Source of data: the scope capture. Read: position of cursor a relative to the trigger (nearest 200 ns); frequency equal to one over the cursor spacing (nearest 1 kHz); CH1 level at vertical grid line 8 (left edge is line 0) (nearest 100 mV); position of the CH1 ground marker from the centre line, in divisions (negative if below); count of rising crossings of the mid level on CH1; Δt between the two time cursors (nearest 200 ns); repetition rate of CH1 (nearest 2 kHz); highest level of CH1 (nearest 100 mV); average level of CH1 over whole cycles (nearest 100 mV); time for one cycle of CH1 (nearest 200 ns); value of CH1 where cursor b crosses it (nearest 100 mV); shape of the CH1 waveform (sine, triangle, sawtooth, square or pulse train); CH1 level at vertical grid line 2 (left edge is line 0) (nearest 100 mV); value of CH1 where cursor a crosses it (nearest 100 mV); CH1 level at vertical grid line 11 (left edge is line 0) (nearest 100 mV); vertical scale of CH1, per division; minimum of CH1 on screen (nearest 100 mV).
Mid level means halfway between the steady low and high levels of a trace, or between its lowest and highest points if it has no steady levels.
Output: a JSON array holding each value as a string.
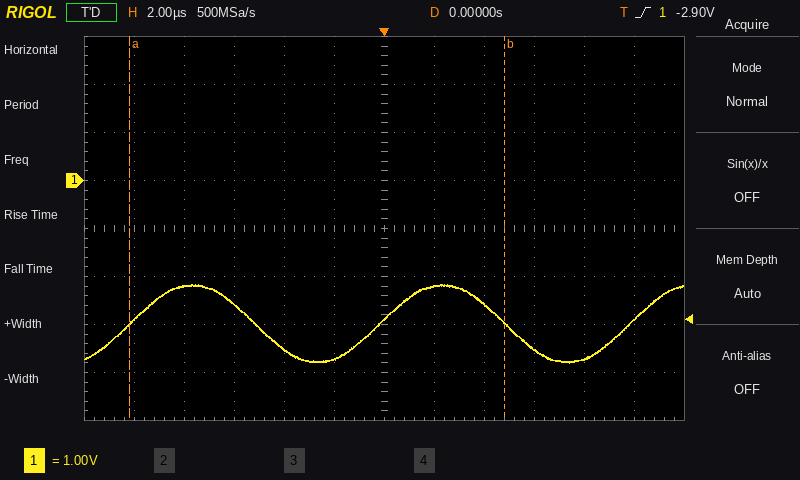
["-10.2 µs", "67 kHz", "-2.6 V", "+1.0 div", "3", "15.0 µs", "100 kHz", "-2.2 V", "-3.0 V", "10.0 µs", "-3.0 V", "sine", "-2.2 V", "-3.0 V", "-2.9 V", "1 V", "-3.8 V"]
